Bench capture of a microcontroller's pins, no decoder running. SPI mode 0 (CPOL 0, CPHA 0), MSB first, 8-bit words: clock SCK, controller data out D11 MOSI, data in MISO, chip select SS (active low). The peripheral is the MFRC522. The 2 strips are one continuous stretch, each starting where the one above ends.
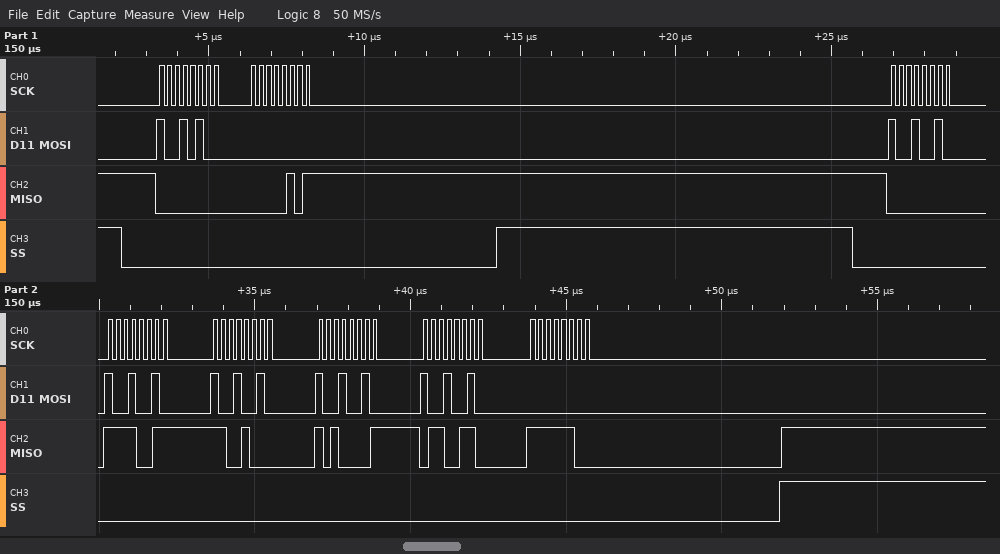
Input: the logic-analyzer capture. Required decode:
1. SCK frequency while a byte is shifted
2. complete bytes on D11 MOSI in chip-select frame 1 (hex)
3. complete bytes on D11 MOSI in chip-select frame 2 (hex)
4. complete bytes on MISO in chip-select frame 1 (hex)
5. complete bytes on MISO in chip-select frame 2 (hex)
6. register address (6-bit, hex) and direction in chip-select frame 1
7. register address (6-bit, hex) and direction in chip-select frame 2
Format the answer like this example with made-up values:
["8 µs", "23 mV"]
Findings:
["4 MHz", "94 00", "92 92 92 92 92 00", "00 05", "00 F3 C8 A1 66 FC", "0x0A read", "0x09 read"]
